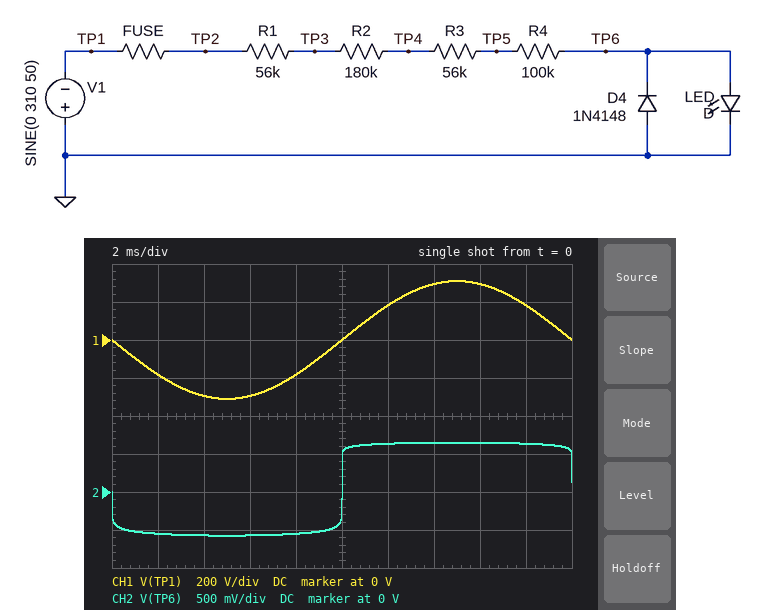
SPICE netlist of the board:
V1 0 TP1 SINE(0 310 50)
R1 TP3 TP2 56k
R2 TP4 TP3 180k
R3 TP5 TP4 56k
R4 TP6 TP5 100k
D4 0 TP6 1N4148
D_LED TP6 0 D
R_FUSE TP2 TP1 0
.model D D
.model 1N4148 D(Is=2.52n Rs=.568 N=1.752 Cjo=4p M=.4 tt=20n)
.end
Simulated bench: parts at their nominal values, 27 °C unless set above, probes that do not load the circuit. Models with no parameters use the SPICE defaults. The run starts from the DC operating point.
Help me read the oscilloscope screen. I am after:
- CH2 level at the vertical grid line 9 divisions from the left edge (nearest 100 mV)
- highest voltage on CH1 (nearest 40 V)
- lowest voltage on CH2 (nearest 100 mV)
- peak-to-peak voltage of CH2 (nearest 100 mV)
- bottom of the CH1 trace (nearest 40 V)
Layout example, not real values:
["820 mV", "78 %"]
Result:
["600 mV", "320 V", "-600 mV", "1.2 V", "-320 V"]
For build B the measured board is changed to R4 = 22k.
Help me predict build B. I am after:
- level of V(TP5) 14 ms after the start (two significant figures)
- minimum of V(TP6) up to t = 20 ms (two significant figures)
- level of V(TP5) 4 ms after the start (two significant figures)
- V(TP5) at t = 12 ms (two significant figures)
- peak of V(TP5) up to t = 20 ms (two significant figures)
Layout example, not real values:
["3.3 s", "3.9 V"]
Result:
["21 V", "-580 mV", "-21 V", "13 V", "22 V"]
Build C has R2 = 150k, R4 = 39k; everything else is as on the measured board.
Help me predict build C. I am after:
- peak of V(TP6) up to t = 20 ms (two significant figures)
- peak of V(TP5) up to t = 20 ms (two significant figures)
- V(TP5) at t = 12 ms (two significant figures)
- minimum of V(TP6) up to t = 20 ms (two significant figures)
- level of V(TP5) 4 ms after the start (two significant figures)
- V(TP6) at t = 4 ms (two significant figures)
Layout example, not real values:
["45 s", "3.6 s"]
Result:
["660 mV", "41 V", "24 V", "-590 mV", "-39 V", "-580 mV"]
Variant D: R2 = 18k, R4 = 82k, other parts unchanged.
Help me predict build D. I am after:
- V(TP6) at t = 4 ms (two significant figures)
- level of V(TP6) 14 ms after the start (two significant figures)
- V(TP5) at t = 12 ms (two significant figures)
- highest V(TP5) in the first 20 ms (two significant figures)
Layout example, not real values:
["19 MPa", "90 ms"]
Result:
["-600 mV", "660 mV", "71 V", "120 V"]
